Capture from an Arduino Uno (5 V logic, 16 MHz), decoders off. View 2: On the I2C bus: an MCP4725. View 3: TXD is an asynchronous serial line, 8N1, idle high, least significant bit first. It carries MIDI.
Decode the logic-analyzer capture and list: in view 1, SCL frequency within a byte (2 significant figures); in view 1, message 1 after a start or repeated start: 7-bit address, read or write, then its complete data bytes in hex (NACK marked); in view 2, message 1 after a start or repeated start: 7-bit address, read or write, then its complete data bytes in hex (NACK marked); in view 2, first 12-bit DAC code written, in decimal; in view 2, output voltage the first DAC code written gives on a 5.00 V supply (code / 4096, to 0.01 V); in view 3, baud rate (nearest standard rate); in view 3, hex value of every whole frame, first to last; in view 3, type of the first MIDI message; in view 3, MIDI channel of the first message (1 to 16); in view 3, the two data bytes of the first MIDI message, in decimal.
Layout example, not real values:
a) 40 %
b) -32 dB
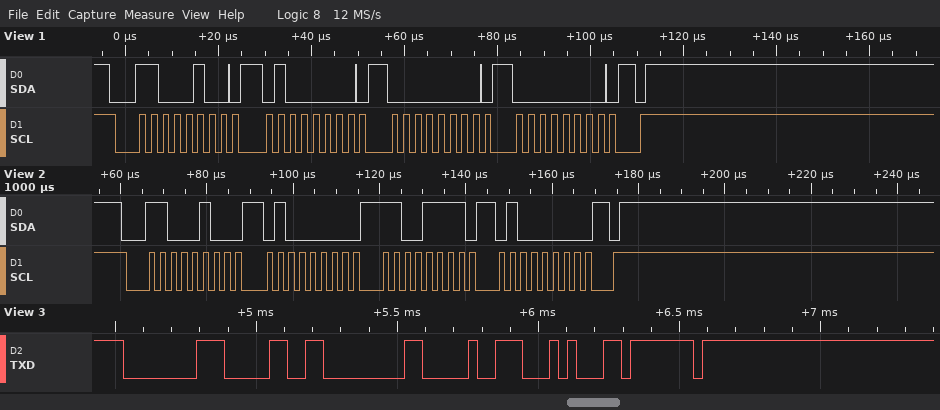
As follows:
a) 400 kHz
b) 0x62 write: 40 00 00
c) 0x62 write: 40 CF 40
d) 3316
e) 4.05 V
f) 31250 baud
g) 80 30 00 90 14 7F
h) Note Off
i) 1
j) 48, 0
